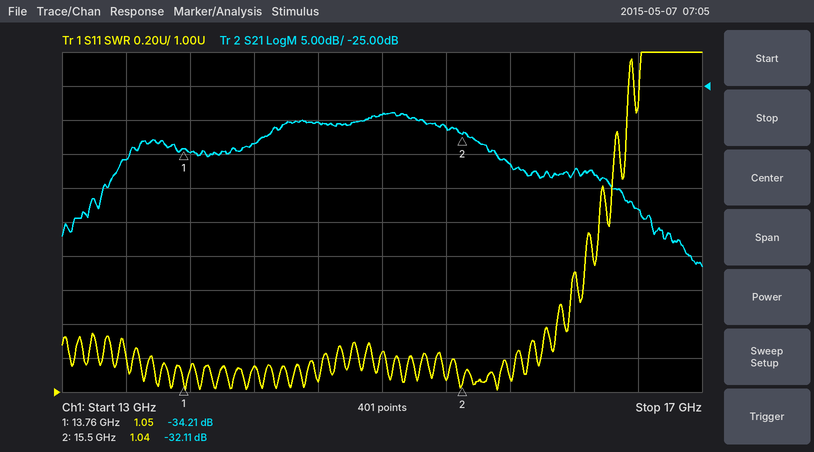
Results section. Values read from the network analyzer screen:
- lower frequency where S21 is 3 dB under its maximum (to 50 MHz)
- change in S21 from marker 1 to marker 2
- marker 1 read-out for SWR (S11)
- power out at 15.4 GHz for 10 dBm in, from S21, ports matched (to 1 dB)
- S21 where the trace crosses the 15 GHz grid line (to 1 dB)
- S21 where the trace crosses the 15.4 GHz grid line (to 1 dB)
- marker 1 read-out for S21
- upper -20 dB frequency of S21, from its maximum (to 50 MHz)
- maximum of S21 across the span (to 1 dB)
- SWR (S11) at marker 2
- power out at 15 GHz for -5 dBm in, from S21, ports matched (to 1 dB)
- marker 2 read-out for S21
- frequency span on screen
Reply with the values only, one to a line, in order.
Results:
14.30 GHz
2.10 dB
1.05
-21 dBm
-29 dB
-31 dB
-34.21 dB
16.90 GHz
-29 dB
1.04
-34 dBm
-32.11 dB
4 GHz
